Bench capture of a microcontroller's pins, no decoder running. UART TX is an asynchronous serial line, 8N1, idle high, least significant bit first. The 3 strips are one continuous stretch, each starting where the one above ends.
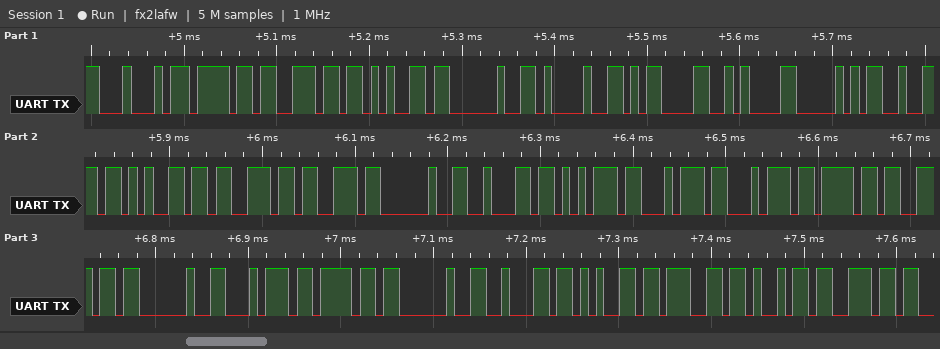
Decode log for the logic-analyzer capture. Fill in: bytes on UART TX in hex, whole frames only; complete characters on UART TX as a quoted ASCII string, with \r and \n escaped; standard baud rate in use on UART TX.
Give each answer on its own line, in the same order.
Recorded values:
44 6F 6E 65 20 21 0D 0A 50 72 65 73 73 20 62 75 74 74 6F 6E 20 74 6F 20 62 65 67 69 6E
"Done !\r\nPress button to begin"
115200 baud
